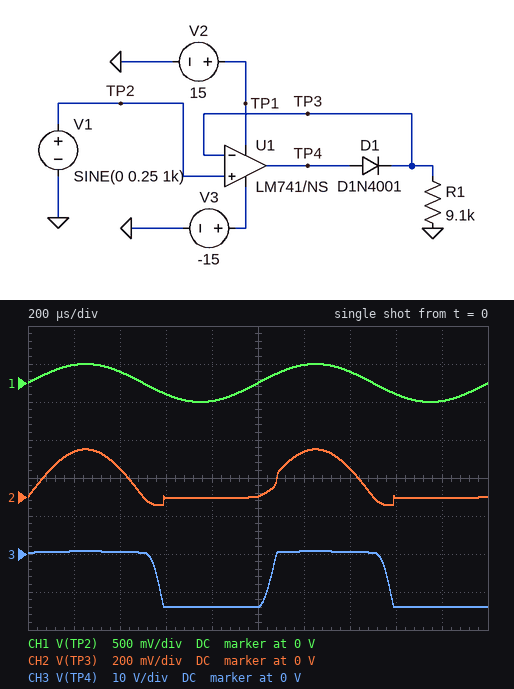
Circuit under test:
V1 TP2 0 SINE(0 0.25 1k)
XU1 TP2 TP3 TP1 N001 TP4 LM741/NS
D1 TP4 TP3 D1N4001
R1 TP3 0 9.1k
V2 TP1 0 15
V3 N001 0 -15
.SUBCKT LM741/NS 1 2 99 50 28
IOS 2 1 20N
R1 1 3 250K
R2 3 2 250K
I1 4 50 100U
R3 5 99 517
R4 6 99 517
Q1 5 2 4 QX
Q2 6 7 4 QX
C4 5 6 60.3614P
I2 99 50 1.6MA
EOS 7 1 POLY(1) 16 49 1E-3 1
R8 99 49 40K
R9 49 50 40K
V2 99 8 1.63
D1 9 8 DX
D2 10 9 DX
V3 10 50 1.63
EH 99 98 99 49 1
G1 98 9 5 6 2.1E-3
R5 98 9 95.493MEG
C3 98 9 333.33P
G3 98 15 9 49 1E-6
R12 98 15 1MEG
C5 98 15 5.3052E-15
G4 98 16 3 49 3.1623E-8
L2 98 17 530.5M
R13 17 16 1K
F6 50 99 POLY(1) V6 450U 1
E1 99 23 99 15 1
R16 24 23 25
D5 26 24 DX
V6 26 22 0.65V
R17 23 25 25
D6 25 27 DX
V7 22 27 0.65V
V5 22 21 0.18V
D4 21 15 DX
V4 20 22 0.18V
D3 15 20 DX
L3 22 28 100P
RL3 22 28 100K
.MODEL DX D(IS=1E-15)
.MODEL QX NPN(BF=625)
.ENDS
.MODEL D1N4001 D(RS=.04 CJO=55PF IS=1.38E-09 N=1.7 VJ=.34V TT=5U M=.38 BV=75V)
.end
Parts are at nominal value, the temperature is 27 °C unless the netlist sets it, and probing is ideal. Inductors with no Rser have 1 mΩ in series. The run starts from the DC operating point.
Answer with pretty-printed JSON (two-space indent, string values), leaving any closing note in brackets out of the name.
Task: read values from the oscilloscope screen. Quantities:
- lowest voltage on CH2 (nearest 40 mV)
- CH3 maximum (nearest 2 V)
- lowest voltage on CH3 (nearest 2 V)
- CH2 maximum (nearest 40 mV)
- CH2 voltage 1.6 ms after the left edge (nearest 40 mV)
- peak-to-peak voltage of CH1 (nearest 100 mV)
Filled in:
{
  "lowest voltage on CH2": "-40 mV",
  "CH3 maximum": "0 V",
  "lowest voltage on CH3": "-14 V",
  "CH2 maximum": "240 mV",
  "CH2 voltage 1.6 ms after the left edge": "0 V",
  "peak-to-peak voltage of CH1": "500 mV"
}
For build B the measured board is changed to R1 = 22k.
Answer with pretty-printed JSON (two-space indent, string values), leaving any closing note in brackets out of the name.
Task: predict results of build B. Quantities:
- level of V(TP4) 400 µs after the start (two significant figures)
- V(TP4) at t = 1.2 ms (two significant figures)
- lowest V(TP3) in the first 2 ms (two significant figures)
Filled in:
{
  "level of V(TP4) 400 µs after the start": "520 mV",
  "V(TP4) at t = 1.2 ms": "630 mV",
  "lowest V(TP3) in the first 2 ms": "-91 mV"
}
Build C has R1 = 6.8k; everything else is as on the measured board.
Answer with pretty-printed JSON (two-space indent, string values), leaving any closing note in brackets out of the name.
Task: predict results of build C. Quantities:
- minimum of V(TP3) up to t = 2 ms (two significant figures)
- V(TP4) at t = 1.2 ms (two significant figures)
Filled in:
{
  "minimum of V(TP3) up to t = 2 ms": "-33 mV",
  "V(TP4) at t = 1.2 ms": "680 mV"
}
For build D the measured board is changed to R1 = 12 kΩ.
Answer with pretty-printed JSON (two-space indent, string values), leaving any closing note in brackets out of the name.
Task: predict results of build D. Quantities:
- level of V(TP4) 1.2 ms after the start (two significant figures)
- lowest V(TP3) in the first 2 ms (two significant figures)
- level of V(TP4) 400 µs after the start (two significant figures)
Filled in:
{
  "level of V(TP4) 1.2 ms after the start": "660 mV",
  "lowest V(TP3) in the first 2 ms": "-54 mV",
  "level of V(TP4) 400 µs after the start": "550 mV"
}
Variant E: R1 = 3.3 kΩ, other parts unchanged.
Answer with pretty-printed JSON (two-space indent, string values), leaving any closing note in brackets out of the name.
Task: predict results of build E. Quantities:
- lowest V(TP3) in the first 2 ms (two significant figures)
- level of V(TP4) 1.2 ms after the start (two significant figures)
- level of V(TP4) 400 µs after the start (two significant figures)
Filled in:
{
  "lowest V(TP3) in the first 2 ms": "-17 mV",
  "level of V(TP4) 1.2 ms after the start": "720 mV",
  "level of V(TP4) 400 µs after the start": "610 mV"
}
